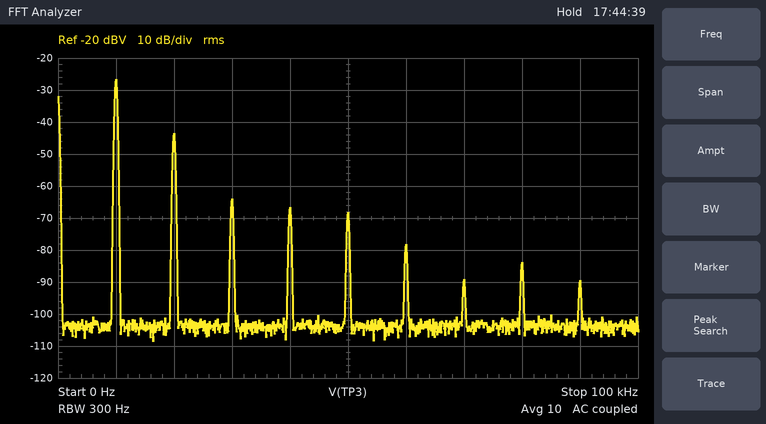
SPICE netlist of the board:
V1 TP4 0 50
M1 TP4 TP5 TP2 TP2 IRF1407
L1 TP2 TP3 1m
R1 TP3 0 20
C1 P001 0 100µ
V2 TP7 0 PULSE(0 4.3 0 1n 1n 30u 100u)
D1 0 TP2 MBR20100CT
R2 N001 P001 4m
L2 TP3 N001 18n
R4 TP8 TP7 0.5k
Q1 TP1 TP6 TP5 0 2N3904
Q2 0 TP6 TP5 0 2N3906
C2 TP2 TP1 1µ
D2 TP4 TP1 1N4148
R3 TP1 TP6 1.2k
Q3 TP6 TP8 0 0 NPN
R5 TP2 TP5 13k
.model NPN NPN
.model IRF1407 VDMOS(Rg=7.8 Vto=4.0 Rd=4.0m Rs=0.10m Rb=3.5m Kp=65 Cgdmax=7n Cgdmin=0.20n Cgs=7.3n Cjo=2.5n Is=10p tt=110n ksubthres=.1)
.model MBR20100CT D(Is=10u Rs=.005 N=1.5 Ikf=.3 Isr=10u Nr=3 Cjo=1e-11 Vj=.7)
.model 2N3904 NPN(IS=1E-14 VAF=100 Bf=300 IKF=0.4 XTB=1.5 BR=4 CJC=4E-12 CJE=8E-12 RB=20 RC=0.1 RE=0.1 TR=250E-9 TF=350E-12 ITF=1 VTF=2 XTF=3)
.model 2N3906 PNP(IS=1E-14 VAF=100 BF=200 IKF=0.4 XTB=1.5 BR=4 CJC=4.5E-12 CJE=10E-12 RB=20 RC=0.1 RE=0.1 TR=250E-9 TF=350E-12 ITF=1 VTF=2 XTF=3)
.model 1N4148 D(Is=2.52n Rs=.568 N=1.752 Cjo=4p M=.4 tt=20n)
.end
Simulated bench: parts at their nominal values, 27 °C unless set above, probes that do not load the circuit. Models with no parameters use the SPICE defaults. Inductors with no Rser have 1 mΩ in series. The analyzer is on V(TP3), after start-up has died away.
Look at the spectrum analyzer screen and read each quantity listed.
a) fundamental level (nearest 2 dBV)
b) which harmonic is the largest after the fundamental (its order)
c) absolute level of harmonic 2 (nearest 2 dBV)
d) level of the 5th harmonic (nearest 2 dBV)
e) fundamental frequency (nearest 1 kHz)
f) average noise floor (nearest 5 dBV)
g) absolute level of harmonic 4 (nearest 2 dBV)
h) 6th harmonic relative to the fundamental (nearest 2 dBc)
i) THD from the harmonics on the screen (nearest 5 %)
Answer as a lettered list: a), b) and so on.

a) -26 dBV
b) 2
c) -44 dBV
d) -68 dBV
e) 10 kHz
f) -105 dBV
g) -66 dBV
h) -52 dBc
i) 15 %
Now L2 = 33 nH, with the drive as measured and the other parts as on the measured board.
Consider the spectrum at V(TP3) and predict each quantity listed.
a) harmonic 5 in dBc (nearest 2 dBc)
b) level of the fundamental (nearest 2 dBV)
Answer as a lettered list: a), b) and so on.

a) -44 dBc
b) -26 dBV
